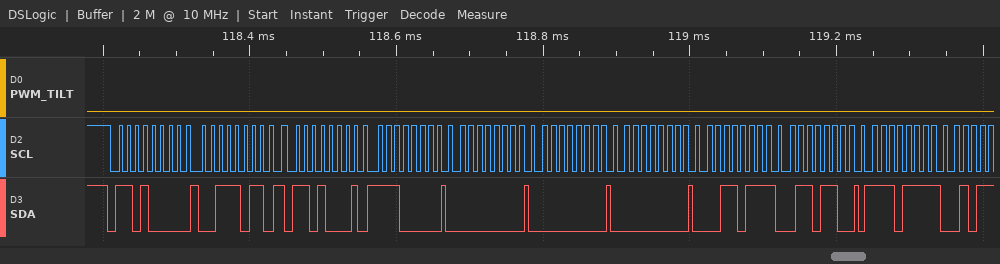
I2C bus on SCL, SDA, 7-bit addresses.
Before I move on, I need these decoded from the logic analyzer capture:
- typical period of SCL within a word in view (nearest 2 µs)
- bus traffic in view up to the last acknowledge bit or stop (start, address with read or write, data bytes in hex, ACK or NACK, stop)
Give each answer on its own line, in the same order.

12 µs
start, address 68 write ACK, 3B ACK, repeated start, address 68 read ACK, E0 ACK, 00 ACK, 00 ACK, 00 ACK, 37 ACK, 6C ACK, EF ACK
